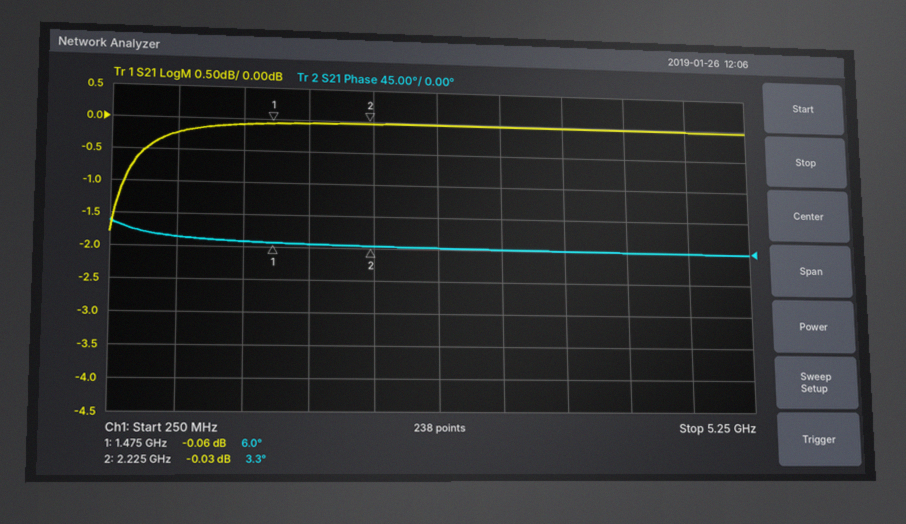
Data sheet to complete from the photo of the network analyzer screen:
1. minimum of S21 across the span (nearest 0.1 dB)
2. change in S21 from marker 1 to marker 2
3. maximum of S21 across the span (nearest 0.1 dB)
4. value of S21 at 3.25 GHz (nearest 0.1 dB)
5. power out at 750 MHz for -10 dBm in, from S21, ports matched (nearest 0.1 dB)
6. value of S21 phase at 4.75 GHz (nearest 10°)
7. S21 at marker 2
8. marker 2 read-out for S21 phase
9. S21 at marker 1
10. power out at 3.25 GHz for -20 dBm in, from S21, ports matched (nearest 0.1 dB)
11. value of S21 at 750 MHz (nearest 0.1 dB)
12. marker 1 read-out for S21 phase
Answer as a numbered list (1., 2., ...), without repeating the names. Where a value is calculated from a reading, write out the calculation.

1. -1.8 dB
2. -0.03 − (-0.06) = 0.03 dB
3. 0.0 dB
4. 0.0 dB
5. -10 dBm + (-0.2 dB) = -10.2 dBm
6. 0°
7. -0.03 dB
8. 3.3°
9. -0.06 dB
10. -20 dBm + (0.0 dB) = -20.0 dBm
11. -0.2 dB
12. 6.0°
